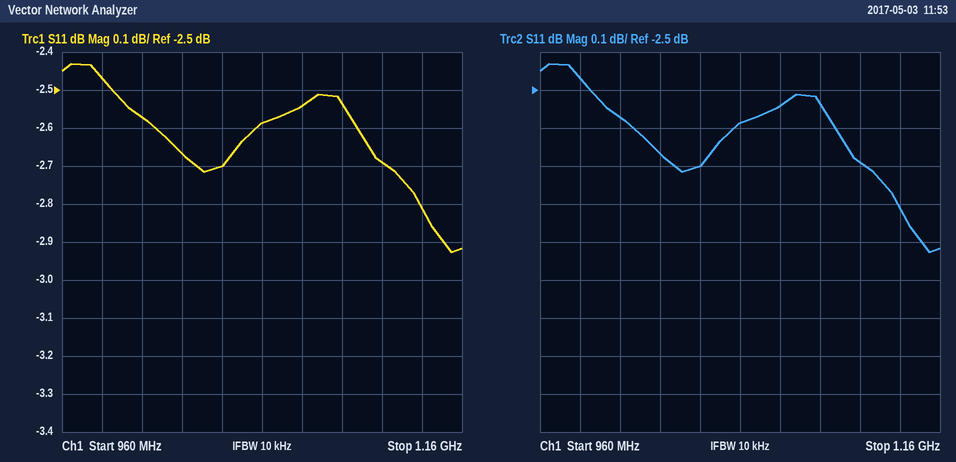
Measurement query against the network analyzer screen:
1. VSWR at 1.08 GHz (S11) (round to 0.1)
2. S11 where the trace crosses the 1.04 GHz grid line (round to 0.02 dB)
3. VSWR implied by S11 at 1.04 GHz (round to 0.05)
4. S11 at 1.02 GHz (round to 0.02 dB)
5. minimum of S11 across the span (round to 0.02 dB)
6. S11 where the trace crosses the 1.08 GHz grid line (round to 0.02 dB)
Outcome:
6.9
-2.70 dB
6.50
-2.66 dB
-2.92 dB
-2.54 dB
